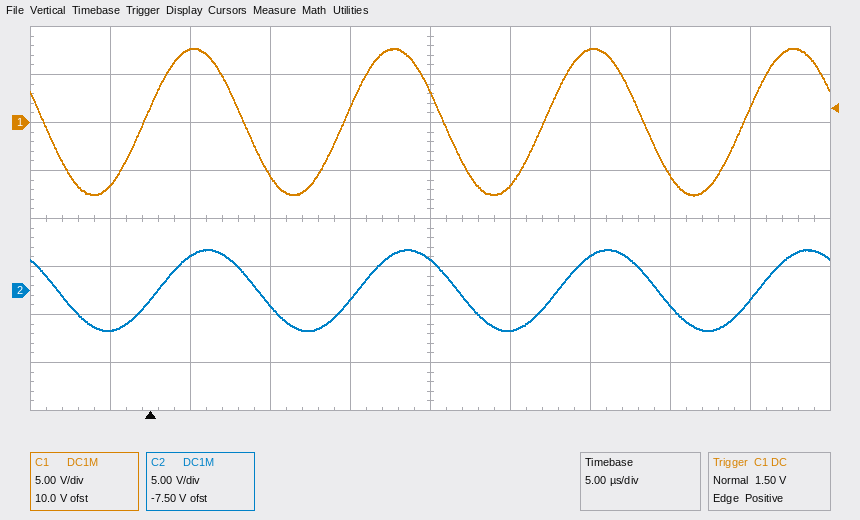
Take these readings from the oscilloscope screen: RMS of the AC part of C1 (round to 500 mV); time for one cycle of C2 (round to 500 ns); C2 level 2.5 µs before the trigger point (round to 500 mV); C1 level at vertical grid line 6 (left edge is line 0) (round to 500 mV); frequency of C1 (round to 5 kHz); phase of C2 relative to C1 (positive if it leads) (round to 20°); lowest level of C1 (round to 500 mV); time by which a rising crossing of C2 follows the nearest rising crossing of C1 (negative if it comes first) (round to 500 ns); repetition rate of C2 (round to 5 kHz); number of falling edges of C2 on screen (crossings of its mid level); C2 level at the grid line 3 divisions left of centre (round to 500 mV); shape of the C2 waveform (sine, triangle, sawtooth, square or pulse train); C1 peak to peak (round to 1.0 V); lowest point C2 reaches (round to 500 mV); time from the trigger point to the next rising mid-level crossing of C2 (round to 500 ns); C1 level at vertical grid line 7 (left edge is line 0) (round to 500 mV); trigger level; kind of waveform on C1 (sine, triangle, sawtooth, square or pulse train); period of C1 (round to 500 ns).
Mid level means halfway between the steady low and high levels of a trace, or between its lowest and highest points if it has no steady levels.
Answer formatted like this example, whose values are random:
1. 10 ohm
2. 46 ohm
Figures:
1. 5.5 V
2. 12.5 µs
3. -4.0 V
4. -6.5 V
5. 80 kHz
6. -20°
7. -7.5 V
8. +1.0 µs
9. 80 kHz
10. 4
11. 3.5 V
12. sine
13. 15.0 V
14. -4.0 V
15. 500 ns
16. 7.5 V
17. 1.50 V
18. sine
19. 12.5 µs
